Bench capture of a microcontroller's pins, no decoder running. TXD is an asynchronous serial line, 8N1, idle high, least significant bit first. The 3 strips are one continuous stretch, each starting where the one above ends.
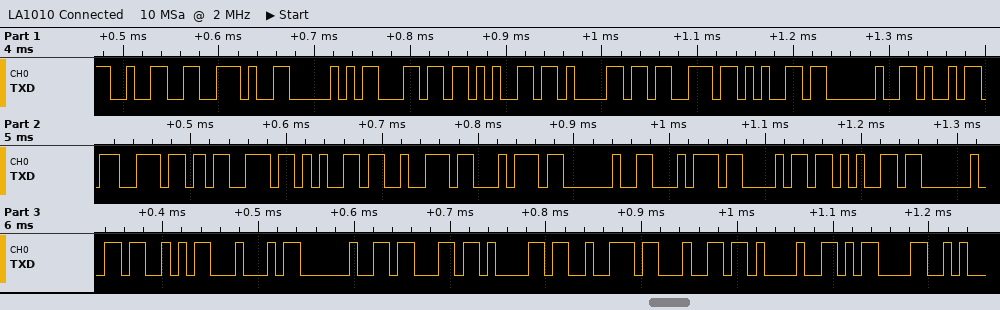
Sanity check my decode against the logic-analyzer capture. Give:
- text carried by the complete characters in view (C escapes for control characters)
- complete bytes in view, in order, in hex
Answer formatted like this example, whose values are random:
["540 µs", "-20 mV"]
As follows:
["\"2.Please insert the SD card!\\r\"", "32 2E 50 6C 65 61 73 65 20 69 6E 73 65 72 74 20 74 68 65 20 53 44 20 63 61 72 64 21 0D"]
